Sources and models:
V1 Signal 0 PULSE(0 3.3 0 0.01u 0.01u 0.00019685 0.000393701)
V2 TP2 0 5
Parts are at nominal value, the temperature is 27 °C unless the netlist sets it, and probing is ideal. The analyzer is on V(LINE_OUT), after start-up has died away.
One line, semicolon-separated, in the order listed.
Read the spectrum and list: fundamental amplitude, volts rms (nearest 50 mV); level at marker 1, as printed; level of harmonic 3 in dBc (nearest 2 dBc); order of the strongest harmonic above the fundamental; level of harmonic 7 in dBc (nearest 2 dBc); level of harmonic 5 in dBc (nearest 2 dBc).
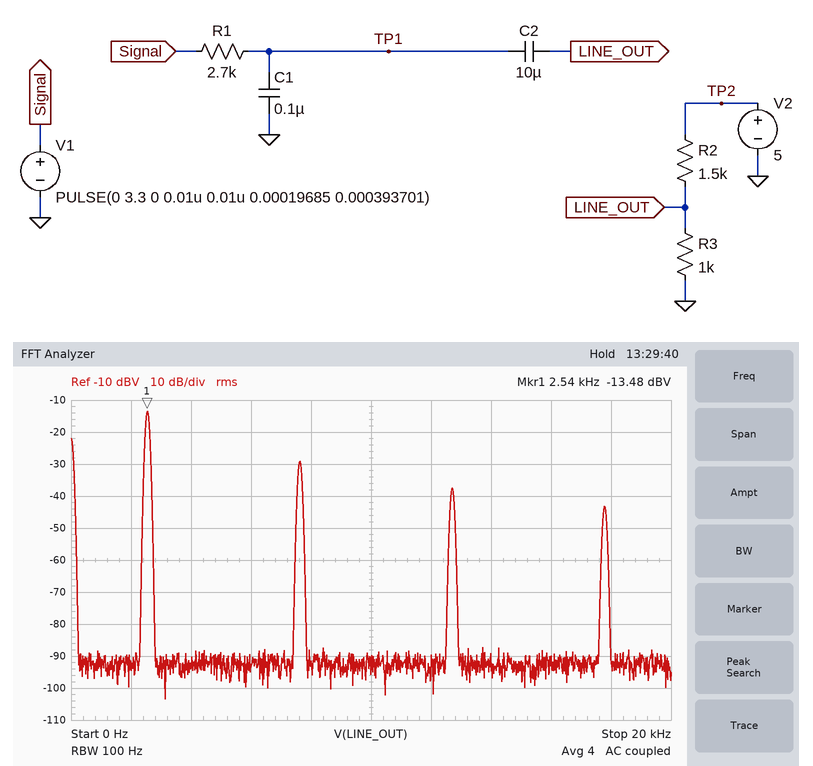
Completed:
200 mV; -13.48 dBV; -16 dBc; 3; -30 dBc; -24 dBc
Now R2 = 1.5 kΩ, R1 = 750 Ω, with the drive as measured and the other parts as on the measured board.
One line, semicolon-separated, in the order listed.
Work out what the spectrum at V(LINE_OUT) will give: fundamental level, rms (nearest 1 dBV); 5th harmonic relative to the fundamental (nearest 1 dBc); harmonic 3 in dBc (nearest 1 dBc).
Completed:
-5 dBV; -22 dBc; -14 dBc
